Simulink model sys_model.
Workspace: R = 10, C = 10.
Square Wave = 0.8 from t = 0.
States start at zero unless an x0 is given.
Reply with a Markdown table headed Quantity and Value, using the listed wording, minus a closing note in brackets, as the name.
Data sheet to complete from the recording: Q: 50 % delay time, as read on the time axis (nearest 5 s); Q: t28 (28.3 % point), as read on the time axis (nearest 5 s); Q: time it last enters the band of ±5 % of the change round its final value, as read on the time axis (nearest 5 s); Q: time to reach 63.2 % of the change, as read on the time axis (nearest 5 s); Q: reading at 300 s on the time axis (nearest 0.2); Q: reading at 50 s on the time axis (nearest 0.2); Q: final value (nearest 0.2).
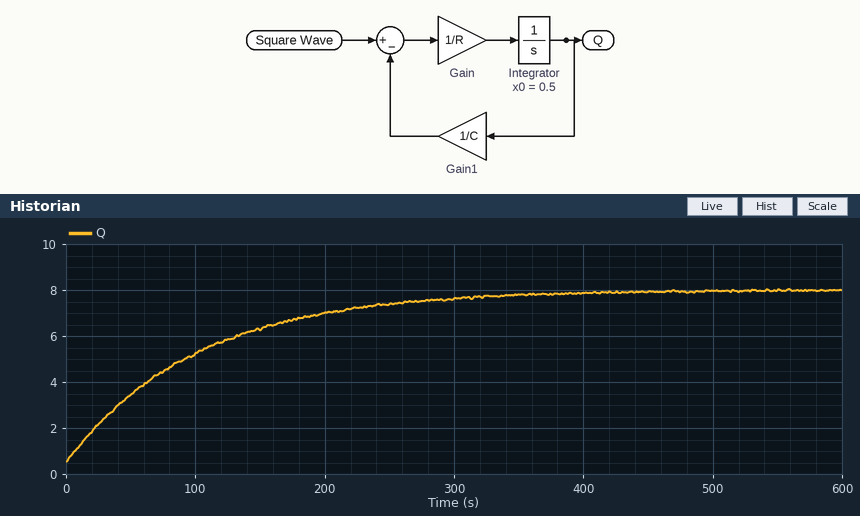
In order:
| Quantity | Value |
|---|---|
| Q: 50 % delay time, as read on the time axis | 70 s |
| Q: t28 (28.3 % point), as read on the time axis | 35 s |
| Q: time it last enters the band of ±5 % of the change round its final value, as read on the time axis | 300 s |
| Q: time to reach 63.2 % of the change, as read on the time axis | 100 s |
| Q: reading at 300 s on the time axis | 7.6 |
| Q: reading at 50 s on the time axis | 3.4 |
| Q: final value | 8.0 |
